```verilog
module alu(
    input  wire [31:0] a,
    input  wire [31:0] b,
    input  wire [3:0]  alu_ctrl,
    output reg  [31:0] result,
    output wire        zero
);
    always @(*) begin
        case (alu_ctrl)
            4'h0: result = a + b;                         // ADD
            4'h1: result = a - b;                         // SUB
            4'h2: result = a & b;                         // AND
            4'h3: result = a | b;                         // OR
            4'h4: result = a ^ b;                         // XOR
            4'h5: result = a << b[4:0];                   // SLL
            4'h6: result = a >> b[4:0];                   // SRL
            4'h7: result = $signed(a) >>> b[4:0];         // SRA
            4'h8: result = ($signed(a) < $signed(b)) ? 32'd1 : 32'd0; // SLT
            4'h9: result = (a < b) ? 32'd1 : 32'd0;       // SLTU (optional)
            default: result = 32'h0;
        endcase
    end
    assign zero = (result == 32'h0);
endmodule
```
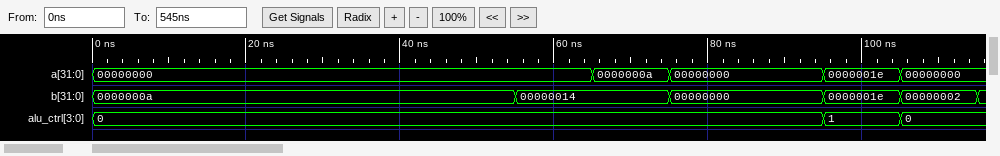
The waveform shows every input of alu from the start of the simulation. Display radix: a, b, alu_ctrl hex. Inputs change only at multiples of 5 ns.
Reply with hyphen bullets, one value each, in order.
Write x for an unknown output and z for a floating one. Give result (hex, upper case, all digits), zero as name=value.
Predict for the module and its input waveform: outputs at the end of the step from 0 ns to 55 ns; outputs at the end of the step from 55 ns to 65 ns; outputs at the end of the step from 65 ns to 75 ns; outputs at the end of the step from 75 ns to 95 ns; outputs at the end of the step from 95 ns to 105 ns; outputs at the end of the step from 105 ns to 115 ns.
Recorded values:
- result=0000000A, zero=0
- result=00000014, zero=0
- result=0000001E, zero=0
- result=00000000, zero=1
- result=00000000, zero=1
- result=00000002, zero=0
